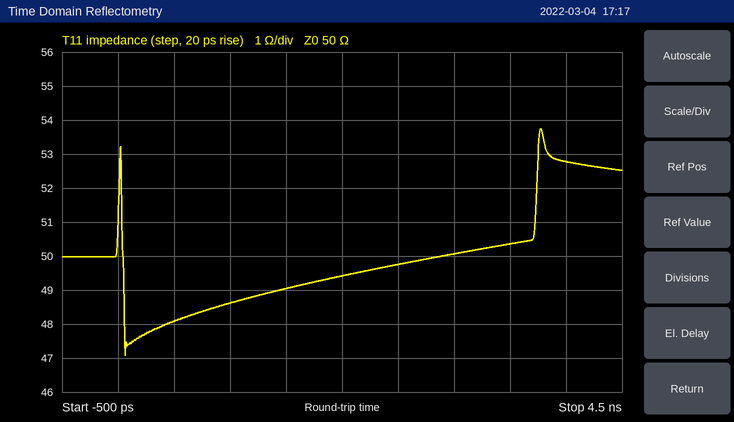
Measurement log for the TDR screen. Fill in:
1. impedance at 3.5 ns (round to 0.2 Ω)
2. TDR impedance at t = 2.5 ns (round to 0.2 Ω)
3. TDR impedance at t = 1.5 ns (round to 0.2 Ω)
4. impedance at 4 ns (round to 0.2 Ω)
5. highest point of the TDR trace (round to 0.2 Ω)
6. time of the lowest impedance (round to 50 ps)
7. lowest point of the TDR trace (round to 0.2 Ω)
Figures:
50.4 Ω
49.8 Ω
49.0 Ω
52.8 Ω
53.8 Ω
50 ps
47.0 Ω
